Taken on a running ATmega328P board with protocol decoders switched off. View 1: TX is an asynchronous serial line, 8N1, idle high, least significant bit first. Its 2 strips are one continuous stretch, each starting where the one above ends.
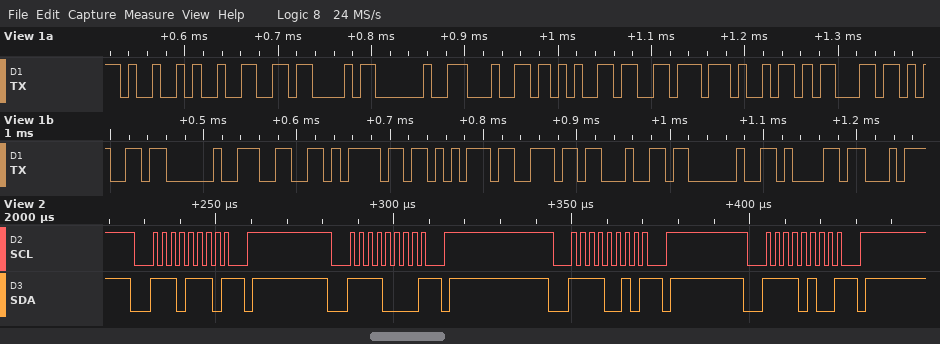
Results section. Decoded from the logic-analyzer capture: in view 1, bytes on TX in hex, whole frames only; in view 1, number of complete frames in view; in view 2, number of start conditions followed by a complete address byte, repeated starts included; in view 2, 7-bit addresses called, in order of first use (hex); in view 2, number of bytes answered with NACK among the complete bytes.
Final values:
49 32 43 20 64 65 76 69 63 65 20 66 6F 75 6E 64 20 61
18
4
0x77 0x78 0x79 0x7A
4
